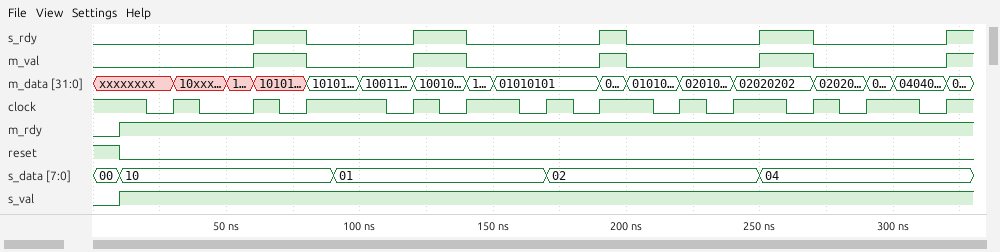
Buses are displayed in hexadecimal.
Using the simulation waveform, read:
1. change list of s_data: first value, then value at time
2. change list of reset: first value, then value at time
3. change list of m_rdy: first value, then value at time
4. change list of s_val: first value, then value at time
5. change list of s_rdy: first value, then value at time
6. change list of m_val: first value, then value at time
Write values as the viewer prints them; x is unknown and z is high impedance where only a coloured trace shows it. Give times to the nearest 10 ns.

00, 10 at 10 ns, 01 at 90 ns, 02 at 170 ns, 04 at 250 ns
1, 0 at 10 ns
0, 1 at 10 ns
0, 1 at 10 ns
0, 1 at 60 ns, 0 at 80 ns, 1 at 120 ns, 0 at 140 ns, 1 at 190 ns, 0 at 200 ns, 1 at 250 ns, 0 at 270 ns, 1 at 320 ns
0, 1 at 60 ns, 0 at 80 ns, 1 at 120 ns, 0 at 140 ns, 1 at 190 ns, 0 at 200 ns, 1 at 250 ns, 0 at 270 ns, 1 at 320 ns
